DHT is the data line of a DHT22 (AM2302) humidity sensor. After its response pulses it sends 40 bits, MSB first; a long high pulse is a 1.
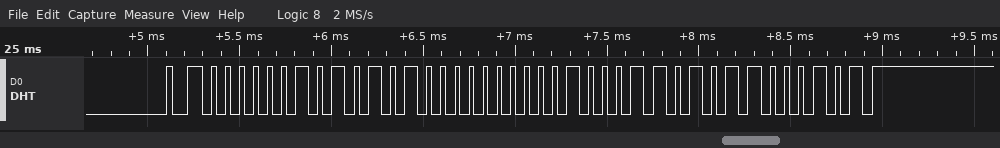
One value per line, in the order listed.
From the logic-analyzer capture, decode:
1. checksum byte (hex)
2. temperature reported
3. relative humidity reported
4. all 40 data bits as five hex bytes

0xC5
28.2 °C
68.0 %
02 A8 01 1A C5
